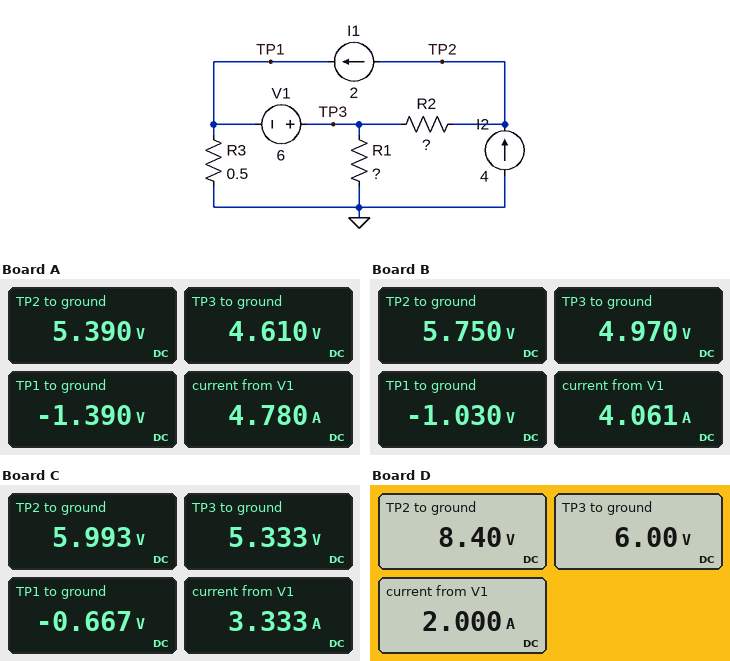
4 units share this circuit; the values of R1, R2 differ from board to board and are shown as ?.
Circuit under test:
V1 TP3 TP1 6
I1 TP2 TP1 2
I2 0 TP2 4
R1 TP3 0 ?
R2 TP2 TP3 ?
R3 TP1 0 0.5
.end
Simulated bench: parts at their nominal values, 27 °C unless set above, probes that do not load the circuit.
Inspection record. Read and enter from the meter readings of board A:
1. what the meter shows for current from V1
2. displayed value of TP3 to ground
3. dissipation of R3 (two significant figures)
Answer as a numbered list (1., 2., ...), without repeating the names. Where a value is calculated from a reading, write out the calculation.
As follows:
1. 4.780 A
2. 4.610 V
3. (0 V - (-1.39 V))^2 / 500 mΩ = 3.9 W
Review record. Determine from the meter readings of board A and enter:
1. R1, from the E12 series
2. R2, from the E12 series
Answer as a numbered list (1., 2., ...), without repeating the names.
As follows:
1. 0.68 Ω
2. 0.39 Ω
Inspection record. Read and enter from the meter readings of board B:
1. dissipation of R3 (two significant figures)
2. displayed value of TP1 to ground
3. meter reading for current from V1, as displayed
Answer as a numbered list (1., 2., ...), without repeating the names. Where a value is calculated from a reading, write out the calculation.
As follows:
1. (0 V - (-1.03 V))^2 / 500 mΩ = 2.1 W
2. -1.030 V
3. 4.061 A
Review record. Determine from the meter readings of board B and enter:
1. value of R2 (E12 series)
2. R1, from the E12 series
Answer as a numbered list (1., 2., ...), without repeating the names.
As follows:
1. 0.39 Ω
2. 0.82 Ω
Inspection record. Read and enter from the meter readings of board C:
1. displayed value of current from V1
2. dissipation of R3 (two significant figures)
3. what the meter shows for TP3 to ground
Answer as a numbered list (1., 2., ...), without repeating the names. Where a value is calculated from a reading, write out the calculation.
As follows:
1. 3.333 A
2. (0 V - (-667 mV))^2 / 500 mΩ = 890 mW
3. 5.333 V
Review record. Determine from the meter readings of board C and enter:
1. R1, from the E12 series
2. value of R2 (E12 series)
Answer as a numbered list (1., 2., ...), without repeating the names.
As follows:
1. 1 Ω
2. 0.33 Ω
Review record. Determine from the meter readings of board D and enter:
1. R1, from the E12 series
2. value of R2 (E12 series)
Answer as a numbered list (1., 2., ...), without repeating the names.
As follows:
1. 1.5 Ω
2. 1.2 Ω
